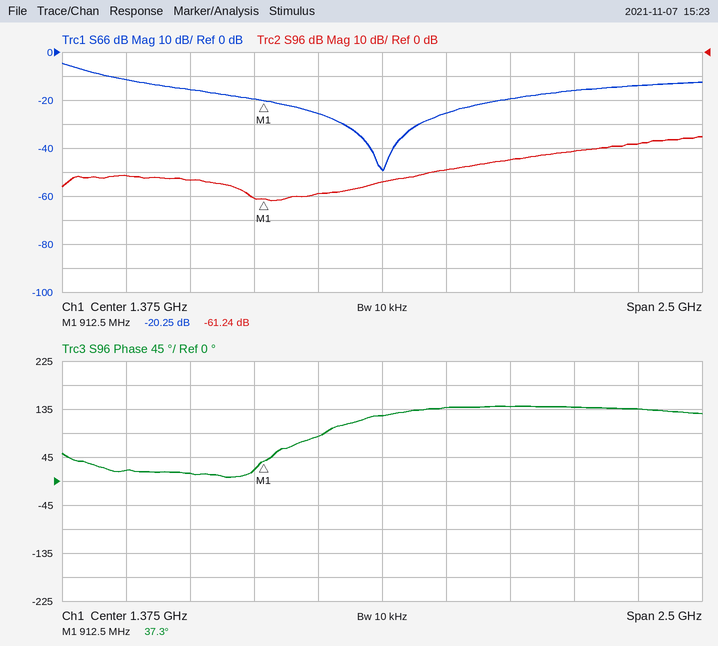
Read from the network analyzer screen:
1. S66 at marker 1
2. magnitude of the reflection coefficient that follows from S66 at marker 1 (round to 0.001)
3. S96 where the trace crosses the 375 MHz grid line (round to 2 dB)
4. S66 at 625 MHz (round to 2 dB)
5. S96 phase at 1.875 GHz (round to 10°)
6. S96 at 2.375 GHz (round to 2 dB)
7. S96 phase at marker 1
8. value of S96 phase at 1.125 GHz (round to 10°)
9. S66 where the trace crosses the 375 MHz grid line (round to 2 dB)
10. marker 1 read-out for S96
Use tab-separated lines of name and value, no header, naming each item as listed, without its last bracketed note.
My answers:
S66 at marker 1	-20.25 dB
magnitude of the reflection coefficient that follows from S66 at marker 1	0.097
S96 where the trace crosses the 375 MHz grid line	-52 dB
S66 at 625 MHz	-16 dB
S96 phase at 1.875 GHz	140°
S96 at 2.375 GHz	-38 dB
S96 phase at marker 1	37.3°
value of S96 phase at 1.125 GHz	80°
S66 where the trace crosses the 375 MHz grid line	-12 dB
marker 1 read-out for S96	-61.24 dB
